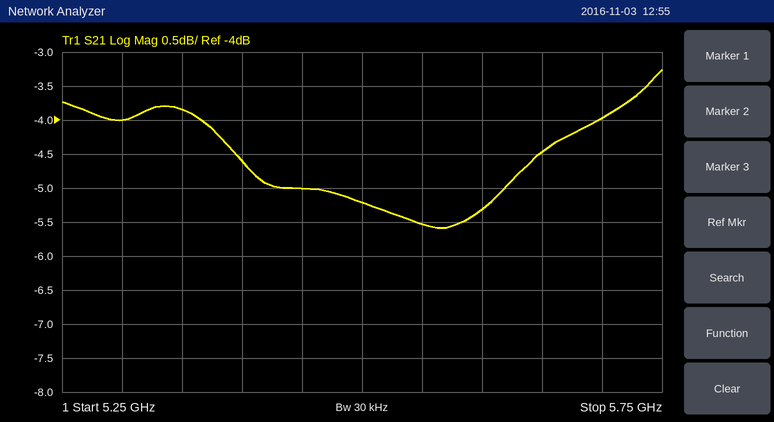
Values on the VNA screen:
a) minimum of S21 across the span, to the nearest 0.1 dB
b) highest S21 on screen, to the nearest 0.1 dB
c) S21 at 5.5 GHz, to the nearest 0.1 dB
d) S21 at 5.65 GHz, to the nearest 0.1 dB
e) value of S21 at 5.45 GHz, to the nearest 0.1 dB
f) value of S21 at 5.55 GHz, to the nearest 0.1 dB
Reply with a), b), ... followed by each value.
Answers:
a) -5.6 dB
b) -3.3 dB
c) -5.2 dB
d) -4.5 dB
e) -5.0 dB
f) -5.5 dB
